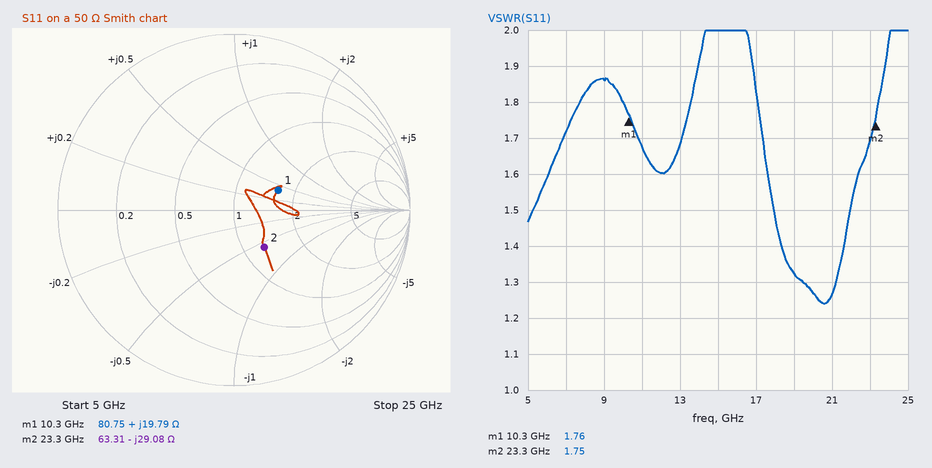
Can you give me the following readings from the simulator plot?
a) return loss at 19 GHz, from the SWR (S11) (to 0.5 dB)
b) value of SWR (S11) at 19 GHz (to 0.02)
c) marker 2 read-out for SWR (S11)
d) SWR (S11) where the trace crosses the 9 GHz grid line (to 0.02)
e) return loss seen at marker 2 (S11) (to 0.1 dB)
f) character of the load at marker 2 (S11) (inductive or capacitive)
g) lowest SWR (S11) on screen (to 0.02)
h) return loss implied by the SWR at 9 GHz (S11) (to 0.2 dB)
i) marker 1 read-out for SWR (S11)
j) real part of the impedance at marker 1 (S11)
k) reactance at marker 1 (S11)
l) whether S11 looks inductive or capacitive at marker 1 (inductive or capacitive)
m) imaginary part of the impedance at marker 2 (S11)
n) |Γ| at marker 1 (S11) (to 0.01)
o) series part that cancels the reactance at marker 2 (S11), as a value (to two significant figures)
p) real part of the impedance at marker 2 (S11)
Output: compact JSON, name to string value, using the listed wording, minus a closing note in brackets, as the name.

{"return loss at 19 GHz, from the SWR (S11)": "17.0 dB", "value of SWR (S11) at 19 GHz": "1.32", "marker 2 read-out for SWR": "1.75", "SWR (S11) where the trace crosses the 9 GHz grid line": "1.86", "return loss seen at marker 2 (S11)": "11.3 dB", "character of the load at marker 2 (S11)": "capacitive", "lowest SWR (S11) on screen": "1.24", "return loss implied by the SWR at 9 GHz (S11)": "10.4 dB", "marker 1 read-out for SWR": "1.76", "real part of the impedance at marker 1": "80.75 Ω", "reactance at marker 1": "+19.79 Ω", "whether S11 looks inductive or capacitive at marker 1": "inductive", "imaginary part of the impedance at marker 2": "-29.08 Ω", "|Γ| at marker 1 (S11)": "0.28", "series part that cancels the reactance at marker 2 (S11), as a value": "200 pH", "real part of the impedance at marker 2": "63.31 Ω"}
